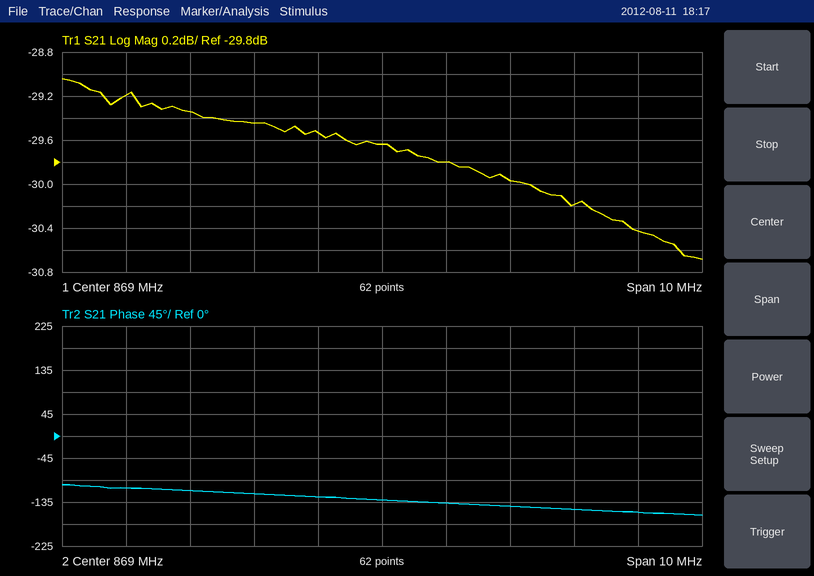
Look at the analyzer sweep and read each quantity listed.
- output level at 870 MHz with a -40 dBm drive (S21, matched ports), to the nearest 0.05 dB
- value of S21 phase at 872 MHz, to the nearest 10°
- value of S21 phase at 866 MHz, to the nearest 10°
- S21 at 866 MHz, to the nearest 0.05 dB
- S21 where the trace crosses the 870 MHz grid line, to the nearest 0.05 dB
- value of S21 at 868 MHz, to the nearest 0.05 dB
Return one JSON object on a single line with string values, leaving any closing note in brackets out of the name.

{"output level at 870 MHz with a -40 dBm drive (S21, matched ports), to the nearest 0.05 dB": "-69.80 dBm", "value of S21 phase at 872 MHz, to the nearest 10°": "-150°", "value of S21 phase at 866 MHz, to the nearest 10°": "-110°", "S21 at 866 MHz, to the nearest 0.05 dB": "-29.35 dB", "S21 where the trace crosses the 870 MHz grid line, to the nearest 0.05 dB": "-29.80 dB", "value of S21 at 868 MHz, to the nearest 0.05 dB": "-29.55 dB"}
